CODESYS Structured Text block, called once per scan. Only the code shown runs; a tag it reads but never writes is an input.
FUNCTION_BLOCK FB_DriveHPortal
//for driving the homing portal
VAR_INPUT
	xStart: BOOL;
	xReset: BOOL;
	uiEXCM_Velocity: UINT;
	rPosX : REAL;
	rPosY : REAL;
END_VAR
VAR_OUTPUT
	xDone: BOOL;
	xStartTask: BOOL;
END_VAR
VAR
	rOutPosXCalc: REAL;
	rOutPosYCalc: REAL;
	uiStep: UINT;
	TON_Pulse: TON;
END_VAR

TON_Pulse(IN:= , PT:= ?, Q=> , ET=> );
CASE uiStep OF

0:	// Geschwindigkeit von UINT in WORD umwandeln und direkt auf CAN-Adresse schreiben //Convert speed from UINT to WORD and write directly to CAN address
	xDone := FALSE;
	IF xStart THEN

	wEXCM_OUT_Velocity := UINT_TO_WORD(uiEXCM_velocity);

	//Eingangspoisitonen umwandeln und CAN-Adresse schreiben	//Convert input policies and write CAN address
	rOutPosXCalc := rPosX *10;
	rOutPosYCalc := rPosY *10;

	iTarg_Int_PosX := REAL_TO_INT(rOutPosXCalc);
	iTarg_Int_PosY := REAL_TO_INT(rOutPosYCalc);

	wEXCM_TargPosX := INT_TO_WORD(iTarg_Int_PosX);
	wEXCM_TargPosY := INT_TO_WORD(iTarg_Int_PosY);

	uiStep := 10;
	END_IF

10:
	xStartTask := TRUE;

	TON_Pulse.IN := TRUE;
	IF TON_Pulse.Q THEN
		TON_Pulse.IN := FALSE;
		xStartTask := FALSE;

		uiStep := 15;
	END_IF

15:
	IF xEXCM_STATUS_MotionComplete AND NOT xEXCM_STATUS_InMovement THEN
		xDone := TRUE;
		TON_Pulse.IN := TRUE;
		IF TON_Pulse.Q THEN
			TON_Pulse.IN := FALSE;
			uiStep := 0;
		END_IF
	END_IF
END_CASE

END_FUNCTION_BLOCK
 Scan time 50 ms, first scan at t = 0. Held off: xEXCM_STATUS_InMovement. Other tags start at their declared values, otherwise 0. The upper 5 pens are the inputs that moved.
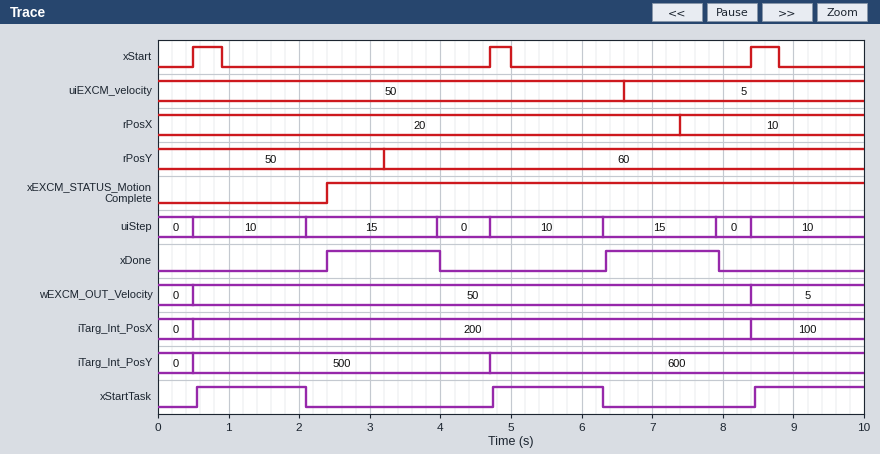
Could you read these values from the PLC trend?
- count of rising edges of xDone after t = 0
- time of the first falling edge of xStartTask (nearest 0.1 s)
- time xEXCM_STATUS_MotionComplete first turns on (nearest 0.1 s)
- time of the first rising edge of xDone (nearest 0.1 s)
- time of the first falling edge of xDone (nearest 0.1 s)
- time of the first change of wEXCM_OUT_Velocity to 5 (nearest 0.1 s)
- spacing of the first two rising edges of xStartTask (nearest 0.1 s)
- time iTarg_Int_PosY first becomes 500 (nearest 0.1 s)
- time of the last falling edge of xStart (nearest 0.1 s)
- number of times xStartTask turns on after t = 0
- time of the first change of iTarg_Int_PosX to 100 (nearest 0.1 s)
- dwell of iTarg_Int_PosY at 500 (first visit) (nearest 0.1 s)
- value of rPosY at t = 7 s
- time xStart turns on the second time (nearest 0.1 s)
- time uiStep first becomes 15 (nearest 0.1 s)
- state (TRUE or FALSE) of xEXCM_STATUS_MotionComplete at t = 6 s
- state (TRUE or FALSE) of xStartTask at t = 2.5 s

2
2.1 s
2.4 s
2.4 s
4.0 s
8.4 s
4.2 s
0.5 s
8.8 s
3
8.4 s
4.2 s
60
4.7 s
2.1 s
TRUE
FALSE
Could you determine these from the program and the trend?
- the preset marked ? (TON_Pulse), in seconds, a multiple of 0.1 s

1.5 s
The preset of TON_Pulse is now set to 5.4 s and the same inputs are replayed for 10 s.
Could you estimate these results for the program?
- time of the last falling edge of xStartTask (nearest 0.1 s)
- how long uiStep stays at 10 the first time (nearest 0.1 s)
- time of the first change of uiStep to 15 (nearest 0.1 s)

6.0 s
5.5 s
6.0 s
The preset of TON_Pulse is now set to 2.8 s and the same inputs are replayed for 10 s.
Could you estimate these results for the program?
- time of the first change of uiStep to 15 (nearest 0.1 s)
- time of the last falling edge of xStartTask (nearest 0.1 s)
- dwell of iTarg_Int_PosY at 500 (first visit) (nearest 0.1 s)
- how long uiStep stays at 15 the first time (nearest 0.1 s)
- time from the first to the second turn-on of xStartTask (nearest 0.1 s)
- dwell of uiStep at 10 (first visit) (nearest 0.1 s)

3.4 s
3.4 s
7.9 s
2.9 s
7.9 s
2.9 s
